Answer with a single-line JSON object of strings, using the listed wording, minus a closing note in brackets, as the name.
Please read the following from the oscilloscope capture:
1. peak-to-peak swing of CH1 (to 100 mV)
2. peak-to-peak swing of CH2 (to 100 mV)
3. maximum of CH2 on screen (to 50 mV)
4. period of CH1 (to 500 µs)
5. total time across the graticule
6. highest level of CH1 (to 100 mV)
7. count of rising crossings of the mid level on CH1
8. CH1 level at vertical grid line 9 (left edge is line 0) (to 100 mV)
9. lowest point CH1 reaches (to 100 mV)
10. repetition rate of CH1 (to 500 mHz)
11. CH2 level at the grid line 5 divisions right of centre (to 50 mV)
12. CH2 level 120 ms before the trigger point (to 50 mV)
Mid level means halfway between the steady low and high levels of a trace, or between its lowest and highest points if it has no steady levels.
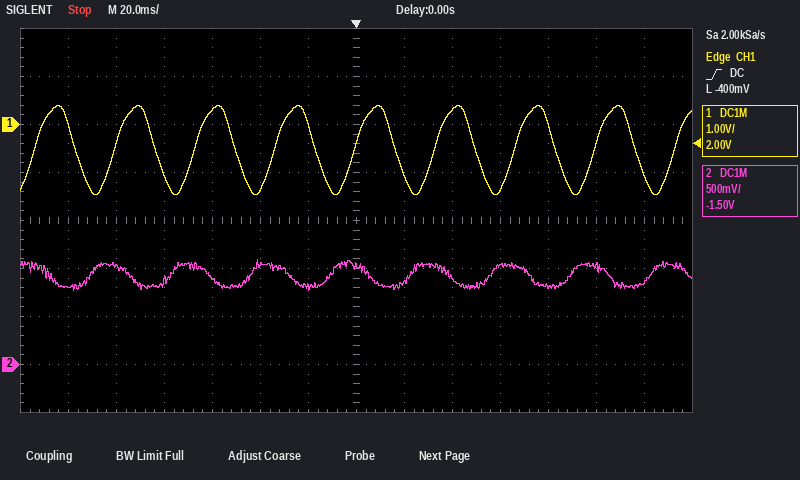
{"peak-to-peak swing of CH1": "1.9 V", "peak-to-peak swing of CH2": "300 mV", "maximum of CH2 on screen": "1.10 V", "period of CH1": "33.5 ms", "total time across the graticule": "280 ms", "highest level of CH1": "400 mV", "count of rising crossings of the mid level on CH1": "9", "CH1 level at vertical grid line 9 (left edge is line 0)": "300 mV", "lowest point CH1 reaches": "-1.5 V", "repetition rate of CH1": "30.0 Hz", "CH2 level at the grid line 5 divisions right of centre": "1.00 V", "CH2 level 120 ms before the trigger point": "800 mV"}
